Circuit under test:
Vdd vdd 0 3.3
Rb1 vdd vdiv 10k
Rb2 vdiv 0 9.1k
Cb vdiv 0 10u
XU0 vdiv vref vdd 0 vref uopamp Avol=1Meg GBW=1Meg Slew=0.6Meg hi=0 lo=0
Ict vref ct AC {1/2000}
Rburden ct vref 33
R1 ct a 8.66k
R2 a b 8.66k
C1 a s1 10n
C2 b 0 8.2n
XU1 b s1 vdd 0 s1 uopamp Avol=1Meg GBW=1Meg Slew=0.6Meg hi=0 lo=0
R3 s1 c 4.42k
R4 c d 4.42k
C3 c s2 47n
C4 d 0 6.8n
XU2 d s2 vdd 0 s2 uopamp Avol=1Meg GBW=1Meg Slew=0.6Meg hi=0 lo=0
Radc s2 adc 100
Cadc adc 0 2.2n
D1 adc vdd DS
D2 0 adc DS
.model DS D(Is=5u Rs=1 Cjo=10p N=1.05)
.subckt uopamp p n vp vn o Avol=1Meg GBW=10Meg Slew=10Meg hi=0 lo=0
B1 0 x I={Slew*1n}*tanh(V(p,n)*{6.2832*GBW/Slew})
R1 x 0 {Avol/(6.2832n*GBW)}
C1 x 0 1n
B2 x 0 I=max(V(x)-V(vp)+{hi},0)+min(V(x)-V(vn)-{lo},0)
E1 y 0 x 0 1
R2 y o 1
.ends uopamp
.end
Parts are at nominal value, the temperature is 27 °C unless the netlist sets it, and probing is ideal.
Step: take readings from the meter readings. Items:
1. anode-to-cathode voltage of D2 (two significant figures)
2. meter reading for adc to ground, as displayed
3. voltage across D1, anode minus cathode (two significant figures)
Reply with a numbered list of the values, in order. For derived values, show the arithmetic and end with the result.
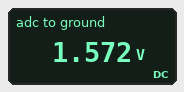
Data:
1. 0 V - 1.572 V = -1.6 V
2. 1.572 V
3. 1.572 V - 3.3 V = -1.7 V
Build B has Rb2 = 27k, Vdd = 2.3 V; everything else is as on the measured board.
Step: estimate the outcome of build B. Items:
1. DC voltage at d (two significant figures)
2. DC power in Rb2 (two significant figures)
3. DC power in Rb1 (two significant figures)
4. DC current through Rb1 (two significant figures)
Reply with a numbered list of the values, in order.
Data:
1. 1.7 V
2. 100 µW
3. 39 µW
4. 62 µA
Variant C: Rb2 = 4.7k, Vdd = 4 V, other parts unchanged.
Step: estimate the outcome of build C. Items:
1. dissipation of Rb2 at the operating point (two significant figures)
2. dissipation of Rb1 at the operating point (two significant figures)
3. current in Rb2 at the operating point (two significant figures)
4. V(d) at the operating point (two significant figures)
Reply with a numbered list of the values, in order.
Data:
1. 350 µW
2. 740 µW
3. 270 µA
4. 1.3 V
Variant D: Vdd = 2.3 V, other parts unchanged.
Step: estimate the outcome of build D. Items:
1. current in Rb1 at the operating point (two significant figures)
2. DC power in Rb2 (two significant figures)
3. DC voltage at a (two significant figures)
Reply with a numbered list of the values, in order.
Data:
1. 120 µA
2. 130 µW
3. 1.1 V
